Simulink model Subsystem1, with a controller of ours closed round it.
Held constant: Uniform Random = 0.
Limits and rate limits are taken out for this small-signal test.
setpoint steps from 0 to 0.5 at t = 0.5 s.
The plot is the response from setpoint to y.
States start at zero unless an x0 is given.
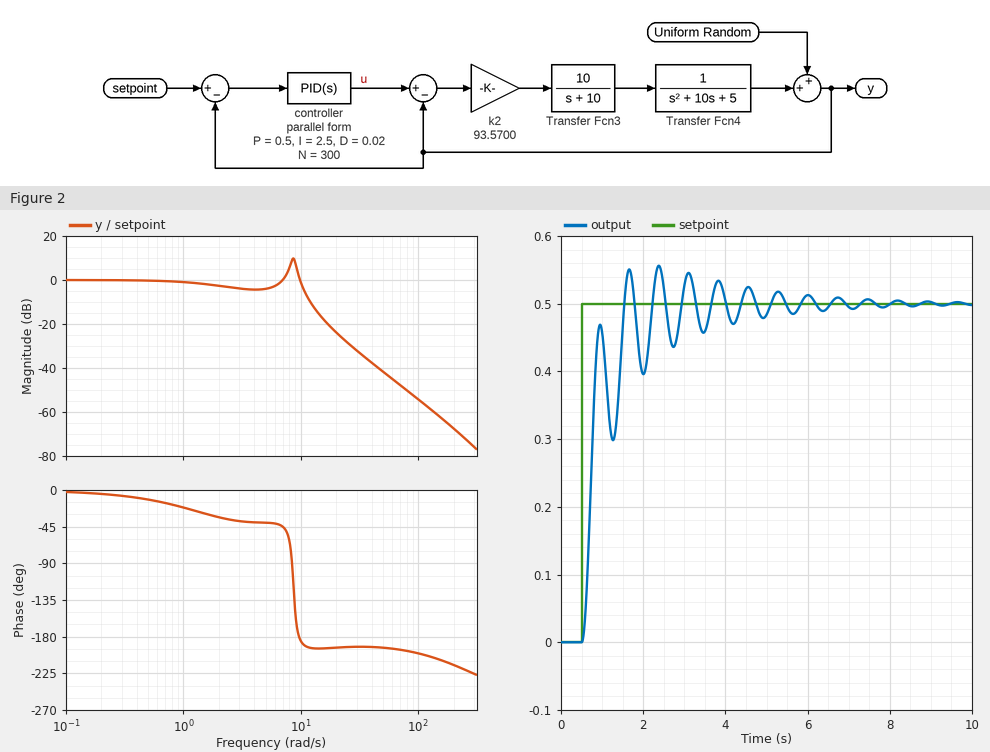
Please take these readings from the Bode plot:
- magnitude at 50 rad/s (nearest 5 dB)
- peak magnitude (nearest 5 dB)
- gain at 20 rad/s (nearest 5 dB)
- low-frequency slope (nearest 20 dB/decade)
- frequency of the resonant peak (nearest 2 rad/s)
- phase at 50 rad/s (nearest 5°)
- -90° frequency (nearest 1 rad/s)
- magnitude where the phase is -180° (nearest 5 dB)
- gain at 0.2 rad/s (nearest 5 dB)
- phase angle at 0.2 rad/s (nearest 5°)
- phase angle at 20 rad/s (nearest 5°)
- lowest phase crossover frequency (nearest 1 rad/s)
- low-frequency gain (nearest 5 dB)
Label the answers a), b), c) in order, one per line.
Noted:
a) -40 dB
b) 10 dB
c) -25 dB
d) 0 dB/decade
e) 8 rad/s
f) -195°
g) 8 rad/s
h) 0 dB
i) 0 dB
j) -5°
k) -195°
l) 10 rad/s
m) 0 dB
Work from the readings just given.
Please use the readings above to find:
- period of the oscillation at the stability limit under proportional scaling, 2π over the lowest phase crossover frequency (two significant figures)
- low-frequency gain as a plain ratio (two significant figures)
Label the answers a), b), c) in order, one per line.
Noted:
a) 0.63 s
b) 1.0
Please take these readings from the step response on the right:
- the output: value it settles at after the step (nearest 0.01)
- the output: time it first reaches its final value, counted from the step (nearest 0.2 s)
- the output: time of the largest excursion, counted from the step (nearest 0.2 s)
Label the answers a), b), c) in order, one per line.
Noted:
a) 0.50
b) 1.0 s
c) 1.8 s
